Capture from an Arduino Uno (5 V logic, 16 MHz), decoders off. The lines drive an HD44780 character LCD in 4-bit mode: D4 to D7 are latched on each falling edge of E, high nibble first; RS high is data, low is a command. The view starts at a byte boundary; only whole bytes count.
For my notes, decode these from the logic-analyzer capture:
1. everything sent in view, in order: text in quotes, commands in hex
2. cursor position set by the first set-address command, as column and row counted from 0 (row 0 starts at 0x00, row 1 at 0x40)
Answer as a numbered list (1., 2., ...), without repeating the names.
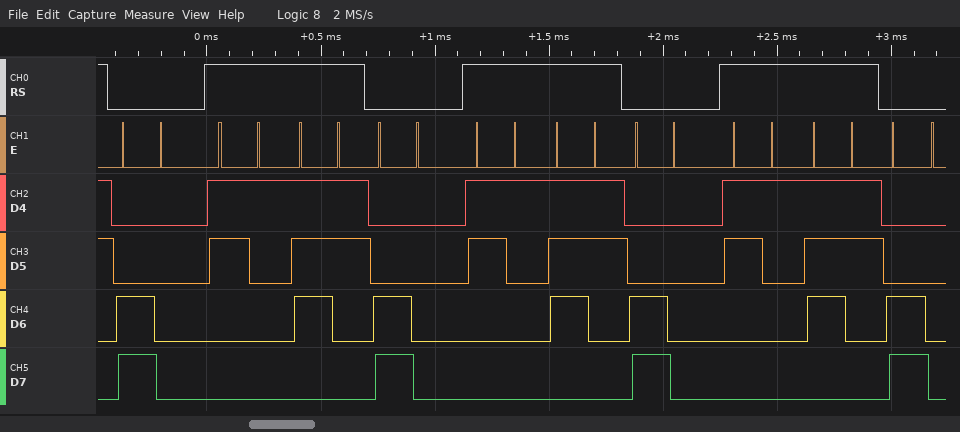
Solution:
1. 0xC0 "1s" 0xC0 "1s" 0xC0 "1s" 0xC0
2. column 0, row 1
